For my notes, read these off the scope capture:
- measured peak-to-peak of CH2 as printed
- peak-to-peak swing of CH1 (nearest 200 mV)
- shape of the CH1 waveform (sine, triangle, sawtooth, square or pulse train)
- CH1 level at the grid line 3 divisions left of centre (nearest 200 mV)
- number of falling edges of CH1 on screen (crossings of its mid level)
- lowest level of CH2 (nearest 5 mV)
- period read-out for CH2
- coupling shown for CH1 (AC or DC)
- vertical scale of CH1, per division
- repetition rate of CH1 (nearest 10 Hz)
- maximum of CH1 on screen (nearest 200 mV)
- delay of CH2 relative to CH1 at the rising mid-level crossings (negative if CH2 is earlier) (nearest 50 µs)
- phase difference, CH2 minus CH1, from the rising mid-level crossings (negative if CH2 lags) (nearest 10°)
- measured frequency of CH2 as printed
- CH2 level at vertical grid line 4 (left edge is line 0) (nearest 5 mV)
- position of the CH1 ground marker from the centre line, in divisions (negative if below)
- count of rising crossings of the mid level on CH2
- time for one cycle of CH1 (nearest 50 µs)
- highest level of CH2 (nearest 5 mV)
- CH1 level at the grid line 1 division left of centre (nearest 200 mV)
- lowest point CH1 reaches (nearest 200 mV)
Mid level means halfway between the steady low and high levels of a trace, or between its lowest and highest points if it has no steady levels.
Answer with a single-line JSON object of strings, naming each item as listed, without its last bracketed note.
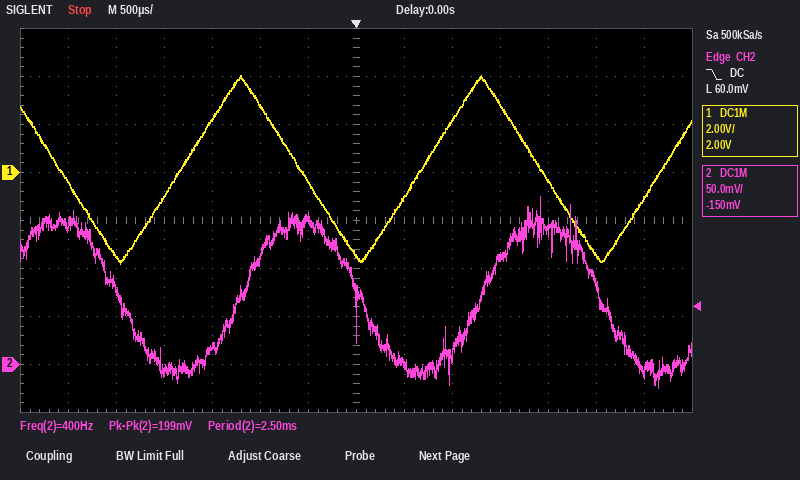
{"measured peak-to-peak of CH2 as printed": "199 mV", "peak-to-peak swing of CH1": "7.8 V", "shape of the CH1 waveform": "triangle", "CH1 level at the grid line 3 divisions left of centre": "2.2 V", "number of falling edges of CH1 on screen": "3", "lowest level of CH2": "-25 mV", "period read-out for CH2": "2.50 ms", "coupling shown for CH1": "DC", "vertical scale of CH1, per division": "2 V", "repetition rate of CH1": "400 Hz", "maximum of CH1 on screen": "4.0 V", "delay of CH2 relative to CH1 at the rising mid-level crossings (negative if CH2 is earlier)": "+650 µs", "phase difference, CH2 minus CH1, from the rising mid-level crossings (negative if CH2 lags)": "-90°", "measured frequency of CH2 as printed": "400 Hz", "CH2 level at vertical grid line 4 (left edge is line 0)": "20 mV", "position of the CH1 ground marker from the centre line, in divisions": "+1.0 div", "count of rising crossings of the mid level on CH2": "2", "time for one cycle of CH1": "2.50 ms", "highest level of CH2": "175 mV", "CH1 level at the grid line 1 division left of centre": "-400 mV", "lowest point CH1 reaches": "-3.8 V"}
